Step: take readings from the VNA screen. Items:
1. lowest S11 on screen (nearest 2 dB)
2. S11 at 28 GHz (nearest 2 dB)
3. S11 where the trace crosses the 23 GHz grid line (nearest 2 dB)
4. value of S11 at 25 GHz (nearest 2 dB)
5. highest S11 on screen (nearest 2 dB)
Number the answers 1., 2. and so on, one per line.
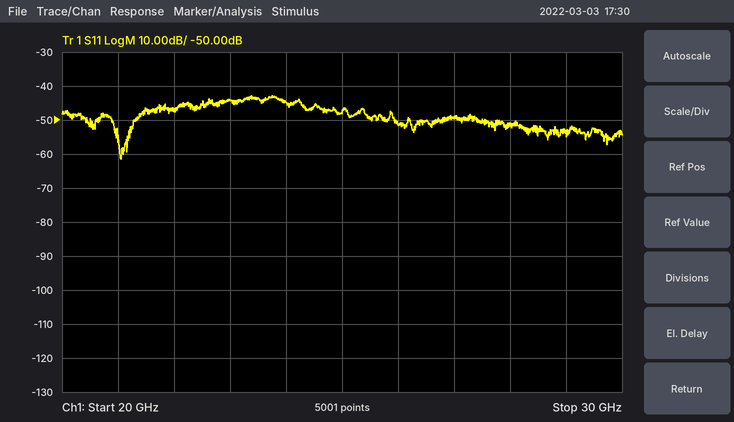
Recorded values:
1. -62 dB
2. -52 dB
3. -44 dB
4. -48 dB
5. -42 dB
